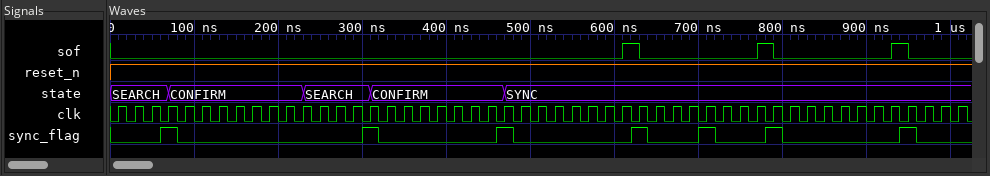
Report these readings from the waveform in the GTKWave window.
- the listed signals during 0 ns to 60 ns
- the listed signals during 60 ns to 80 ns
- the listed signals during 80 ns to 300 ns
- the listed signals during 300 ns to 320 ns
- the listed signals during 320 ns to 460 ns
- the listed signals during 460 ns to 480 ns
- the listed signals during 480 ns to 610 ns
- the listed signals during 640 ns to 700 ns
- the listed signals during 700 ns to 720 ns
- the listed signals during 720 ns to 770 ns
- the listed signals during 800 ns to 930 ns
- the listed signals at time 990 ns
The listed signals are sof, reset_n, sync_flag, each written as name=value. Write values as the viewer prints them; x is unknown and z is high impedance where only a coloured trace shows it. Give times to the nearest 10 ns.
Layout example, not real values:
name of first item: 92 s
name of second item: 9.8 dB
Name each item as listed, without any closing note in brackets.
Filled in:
the listed signals during 0 ns to 60 ns: sof=0, reset_n=1, sync_flag=0
the listed signals during 60 ns to 80 ns: sof=0, reset_n=1, sync_flag=1
the listed signals during 80 ns to 300 ns: sof=0, reset_n=1, sync_flag=0
the listed signals during 300 ns to 320 ns: sof=0, reset_n=1, sync_flag=1
the listed signals during 320 ns to 460 ns: sof=0, reset_n=1, sync_flag=0
the listed signals during 460 ns to 480 ns: sof=0, reset_n=1, sync_flag=1
the listed signals during 480 ns to 610 ns: sof=0, reset_n=1, sync_flag=0
the listed signals during 640 ns to 700 ns: sof=0, reset_n=1, sync_flag=0
the listed signals during 700 ns to 720 ns: sof=0, reset_n=1, sync_flag=1
the listed signals during 720 ns to 770 ns: sof=0, reset_n=1, sync_flag=0
the listed signals during 800 ns to 930 ns: sof=0, reset_n=1, sync_flag=0
the listed signals at time 990 ns: sof=0, reset_n=1, sync_flag=0
